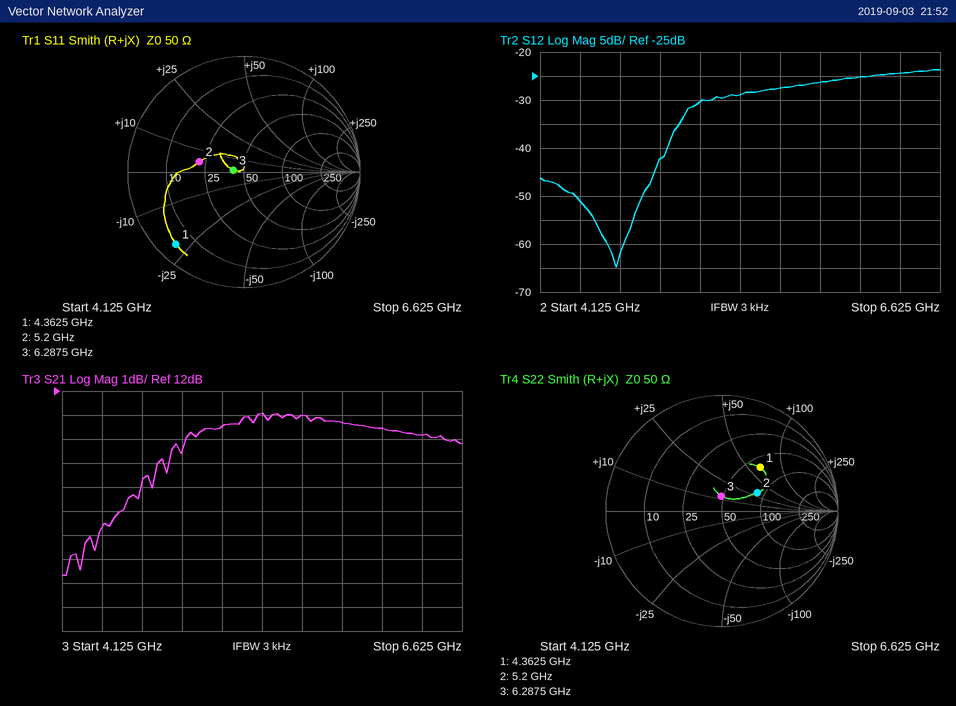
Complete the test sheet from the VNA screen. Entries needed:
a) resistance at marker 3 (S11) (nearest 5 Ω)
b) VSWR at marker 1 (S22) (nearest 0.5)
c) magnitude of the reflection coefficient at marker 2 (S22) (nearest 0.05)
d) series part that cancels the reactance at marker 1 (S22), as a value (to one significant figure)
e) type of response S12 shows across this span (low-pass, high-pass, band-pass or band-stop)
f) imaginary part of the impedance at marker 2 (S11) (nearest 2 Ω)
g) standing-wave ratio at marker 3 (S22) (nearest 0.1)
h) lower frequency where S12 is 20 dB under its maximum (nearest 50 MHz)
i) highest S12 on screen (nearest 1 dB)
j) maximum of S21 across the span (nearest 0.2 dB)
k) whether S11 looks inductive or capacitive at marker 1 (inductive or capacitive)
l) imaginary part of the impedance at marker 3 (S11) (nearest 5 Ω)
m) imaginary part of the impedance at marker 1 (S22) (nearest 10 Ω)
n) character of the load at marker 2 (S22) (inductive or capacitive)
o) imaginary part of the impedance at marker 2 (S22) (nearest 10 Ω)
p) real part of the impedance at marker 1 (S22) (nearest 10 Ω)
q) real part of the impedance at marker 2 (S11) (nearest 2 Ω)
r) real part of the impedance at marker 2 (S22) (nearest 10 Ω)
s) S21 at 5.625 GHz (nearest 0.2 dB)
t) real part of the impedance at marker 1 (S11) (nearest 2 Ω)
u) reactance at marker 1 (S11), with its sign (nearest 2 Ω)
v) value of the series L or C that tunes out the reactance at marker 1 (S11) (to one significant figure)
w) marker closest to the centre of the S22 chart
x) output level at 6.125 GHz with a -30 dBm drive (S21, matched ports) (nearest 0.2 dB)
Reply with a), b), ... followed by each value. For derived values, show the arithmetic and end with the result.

a) 40 Ω
b) 3.0
c) 0.35
d) C = 1/(2π × 4.3625 GHz × 60 Ω) ≈ 608 fF, so 600 fF to one significant figure
e) high-pass
f) +4 Ω
g) 1.3
h) 4.85 GHz
i) -24 dB
j) 11.0 dB
k) capacitive
l) 0 Ω
m) +60 Ω
n) inductive
o) +30 Ω
p) 60 Ω
q) 22 Ω
r) 90 Ω
s) 11.0 dB
t) 4 Ω
u) -22 Ω
v) L = 22 Ω/(2π × 4.3625 GHz) ≈ 803 pH, so 800 pH to one significant figure
w) marker 3
x) -30 dBm + (10.4 dB) = -19.6 dBm
